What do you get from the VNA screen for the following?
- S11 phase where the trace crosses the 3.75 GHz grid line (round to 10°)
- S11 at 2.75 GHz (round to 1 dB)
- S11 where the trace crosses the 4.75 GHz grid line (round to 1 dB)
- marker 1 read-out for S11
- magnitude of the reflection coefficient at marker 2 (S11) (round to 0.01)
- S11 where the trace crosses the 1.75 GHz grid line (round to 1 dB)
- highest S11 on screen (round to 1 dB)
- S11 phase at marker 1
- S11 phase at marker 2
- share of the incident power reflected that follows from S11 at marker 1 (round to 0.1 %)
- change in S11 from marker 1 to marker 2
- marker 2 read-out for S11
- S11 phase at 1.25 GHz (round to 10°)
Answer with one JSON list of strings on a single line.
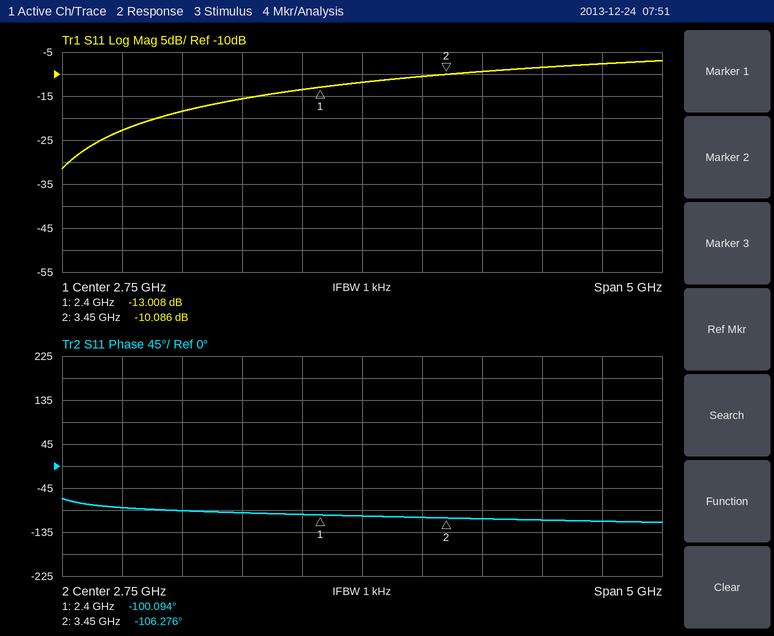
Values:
["-110°", "-12 dB", "-8 dB", "-13.008 dB", "0.31", "-16 dB", "-7 dB", "-100.094°", "-106.276°", "5.0 %", "2.922 dB", "-10.086 dB", "-90°"]
